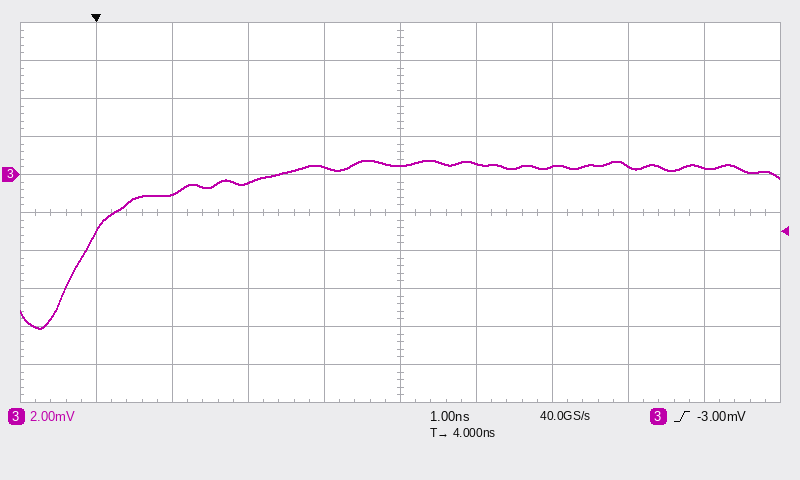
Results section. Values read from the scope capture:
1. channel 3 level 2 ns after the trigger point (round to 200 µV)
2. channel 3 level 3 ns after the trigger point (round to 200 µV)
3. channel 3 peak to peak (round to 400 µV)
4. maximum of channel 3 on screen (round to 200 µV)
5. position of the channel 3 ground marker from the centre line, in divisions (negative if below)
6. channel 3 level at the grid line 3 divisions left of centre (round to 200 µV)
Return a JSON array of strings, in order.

["-400 µV", "400 µV", "8.8 mV", "800 µV", "+1.0 div", "-1.0 mV"]
